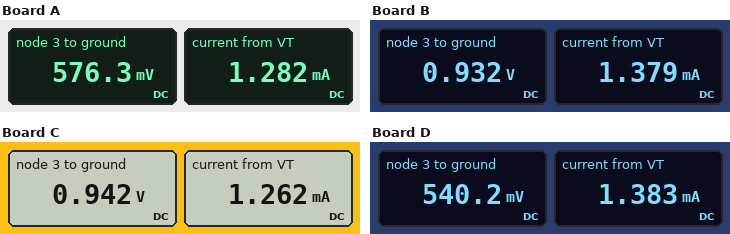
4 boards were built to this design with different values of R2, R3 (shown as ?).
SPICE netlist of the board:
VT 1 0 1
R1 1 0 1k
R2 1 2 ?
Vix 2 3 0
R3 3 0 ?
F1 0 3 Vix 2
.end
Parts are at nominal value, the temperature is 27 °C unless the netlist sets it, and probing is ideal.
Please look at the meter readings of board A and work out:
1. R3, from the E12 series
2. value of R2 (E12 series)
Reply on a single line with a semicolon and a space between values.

680 Ω; 1.5 kΩ
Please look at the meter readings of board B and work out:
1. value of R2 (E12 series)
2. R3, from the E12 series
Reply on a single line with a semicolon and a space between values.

180 Ω; 820 Ω
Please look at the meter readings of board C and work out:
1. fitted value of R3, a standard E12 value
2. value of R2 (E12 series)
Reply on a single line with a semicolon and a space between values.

1.2 kΩ; 220 Ω
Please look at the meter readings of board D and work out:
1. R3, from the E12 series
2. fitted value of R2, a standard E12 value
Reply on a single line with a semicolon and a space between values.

470 Ω; 1.2 kΩ
